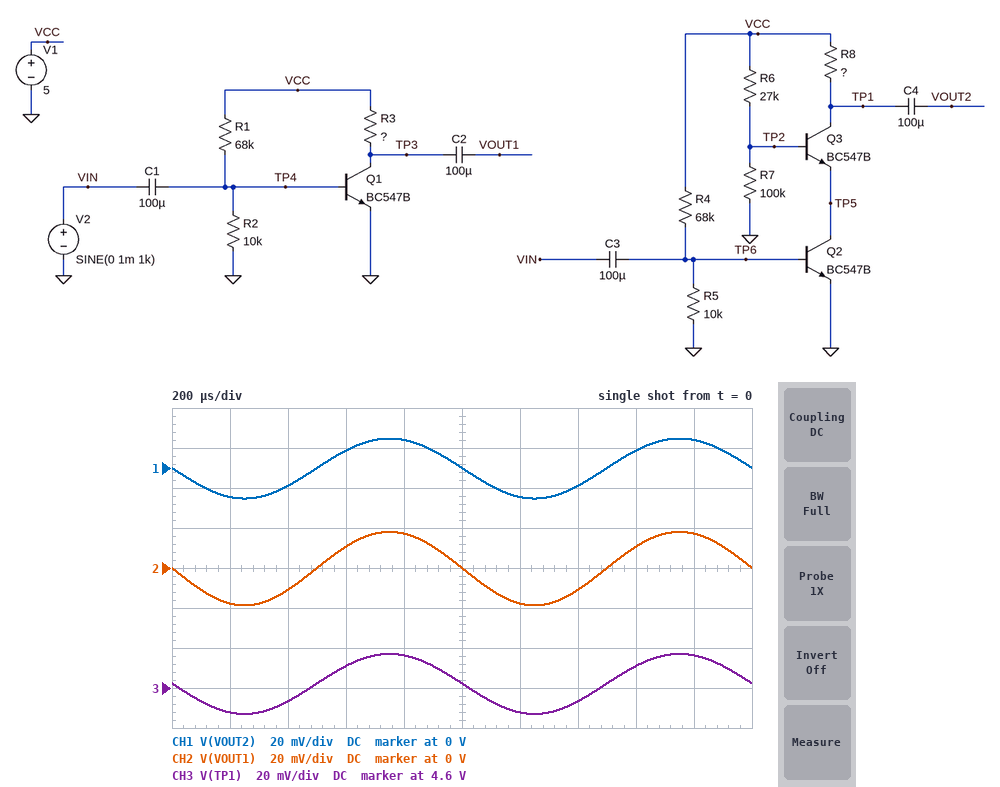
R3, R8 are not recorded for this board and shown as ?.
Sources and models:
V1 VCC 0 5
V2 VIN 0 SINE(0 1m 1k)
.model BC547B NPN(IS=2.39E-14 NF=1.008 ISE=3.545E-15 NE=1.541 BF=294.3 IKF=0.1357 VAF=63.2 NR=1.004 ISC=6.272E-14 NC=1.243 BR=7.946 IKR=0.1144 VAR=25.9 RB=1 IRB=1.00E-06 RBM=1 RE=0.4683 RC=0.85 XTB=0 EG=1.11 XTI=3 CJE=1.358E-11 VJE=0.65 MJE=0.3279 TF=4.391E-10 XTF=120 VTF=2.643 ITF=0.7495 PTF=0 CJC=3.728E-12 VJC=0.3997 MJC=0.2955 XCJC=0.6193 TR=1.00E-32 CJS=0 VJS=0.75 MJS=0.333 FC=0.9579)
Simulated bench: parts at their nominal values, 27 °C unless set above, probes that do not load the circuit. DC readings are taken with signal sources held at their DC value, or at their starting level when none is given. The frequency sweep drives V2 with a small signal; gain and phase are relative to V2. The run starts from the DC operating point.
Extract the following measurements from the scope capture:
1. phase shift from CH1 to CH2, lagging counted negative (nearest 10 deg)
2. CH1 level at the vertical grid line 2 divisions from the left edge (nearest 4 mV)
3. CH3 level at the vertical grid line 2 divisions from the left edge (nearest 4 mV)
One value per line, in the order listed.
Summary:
0 deg
-8 mV
4.592 V
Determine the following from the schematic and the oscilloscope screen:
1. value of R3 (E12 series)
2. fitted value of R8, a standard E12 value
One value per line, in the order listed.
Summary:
820 Ω
680 Ω
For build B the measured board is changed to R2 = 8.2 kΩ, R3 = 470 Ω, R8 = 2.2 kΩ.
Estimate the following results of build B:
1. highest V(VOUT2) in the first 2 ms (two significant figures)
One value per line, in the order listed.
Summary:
48 mV
